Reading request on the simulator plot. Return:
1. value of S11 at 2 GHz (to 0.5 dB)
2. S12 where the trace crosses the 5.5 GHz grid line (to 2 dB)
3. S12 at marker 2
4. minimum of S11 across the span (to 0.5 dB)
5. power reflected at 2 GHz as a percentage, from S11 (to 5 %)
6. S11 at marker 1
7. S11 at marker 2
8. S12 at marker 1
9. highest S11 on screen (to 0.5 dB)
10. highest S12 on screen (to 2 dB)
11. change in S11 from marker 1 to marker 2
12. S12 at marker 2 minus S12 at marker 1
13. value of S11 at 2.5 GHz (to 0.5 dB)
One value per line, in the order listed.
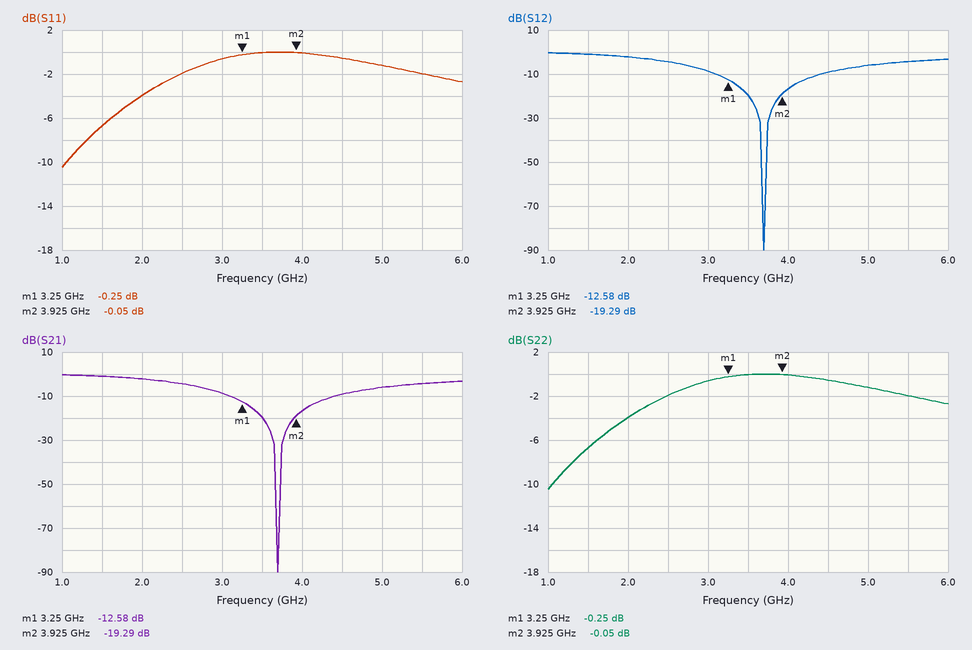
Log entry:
-4.0 dB
-4 dB
-19.29 dB
-10.5 dB
40 %
-0.25 dB
-0.05 dB
-12.58 dB
0.0 dB
0 dB
0.20 dB
-6.71 dB
-2.0 dB
